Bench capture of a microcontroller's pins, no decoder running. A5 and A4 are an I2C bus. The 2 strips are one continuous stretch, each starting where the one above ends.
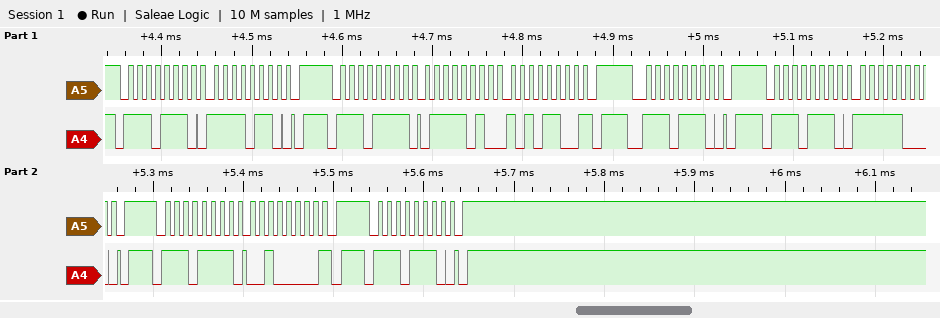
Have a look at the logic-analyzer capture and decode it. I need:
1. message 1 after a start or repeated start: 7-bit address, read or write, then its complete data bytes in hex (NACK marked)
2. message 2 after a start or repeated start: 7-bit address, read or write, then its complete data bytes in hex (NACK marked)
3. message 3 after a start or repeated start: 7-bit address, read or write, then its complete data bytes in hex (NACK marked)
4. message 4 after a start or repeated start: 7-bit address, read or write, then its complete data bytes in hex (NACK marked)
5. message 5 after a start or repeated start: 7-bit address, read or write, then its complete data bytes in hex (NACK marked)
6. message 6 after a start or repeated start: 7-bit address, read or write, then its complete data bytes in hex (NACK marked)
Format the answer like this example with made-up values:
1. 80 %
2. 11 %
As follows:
1. 0x77 write: F6
2. 0x77 read: 7A AC NACK
3. 0x77 write
4. 0x77 write: F8
5. 0x77 read: 20 NACK
6. 0x77 write
